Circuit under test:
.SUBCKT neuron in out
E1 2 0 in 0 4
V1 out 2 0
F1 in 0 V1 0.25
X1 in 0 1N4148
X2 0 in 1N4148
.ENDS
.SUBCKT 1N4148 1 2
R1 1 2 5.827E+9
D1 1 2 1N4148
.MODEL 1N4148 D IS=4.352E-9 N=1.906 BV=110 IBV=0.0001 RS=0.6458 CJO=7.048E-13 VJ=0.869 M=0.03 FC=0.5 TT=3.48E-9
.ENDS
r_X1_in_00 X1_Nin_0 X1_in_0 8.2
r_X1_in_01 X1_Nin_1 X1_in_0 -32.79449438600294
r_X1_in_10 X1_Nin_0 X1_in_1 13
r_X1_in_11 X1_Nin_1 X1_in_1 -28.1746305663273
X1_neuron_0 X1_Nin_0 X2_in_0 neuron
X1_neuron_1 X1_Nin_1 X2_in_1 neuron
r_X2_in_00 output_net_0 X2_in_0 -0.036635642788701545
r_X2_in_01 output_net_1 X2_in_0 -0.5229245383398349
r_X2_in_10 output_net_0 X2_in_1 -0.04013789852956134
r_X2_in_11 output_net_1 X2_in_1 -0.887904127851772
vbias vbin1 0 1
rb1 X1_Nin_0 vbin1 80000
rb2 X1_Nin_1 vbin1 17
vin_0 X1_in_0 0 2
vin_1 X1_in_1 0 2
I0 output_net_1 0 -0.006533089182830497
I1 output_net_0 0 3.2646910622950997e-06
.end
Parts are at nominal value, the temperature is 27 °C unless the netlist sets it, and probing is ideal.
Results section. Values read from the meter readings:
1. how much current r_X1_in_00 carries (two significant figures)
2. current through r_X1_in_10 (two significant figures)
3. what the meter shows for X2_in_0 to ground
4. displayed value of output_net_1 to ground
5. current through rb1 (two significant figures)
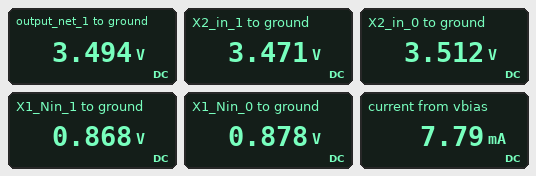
140 mA
86 mA
3.512 V
3.494 V
1.5 µA
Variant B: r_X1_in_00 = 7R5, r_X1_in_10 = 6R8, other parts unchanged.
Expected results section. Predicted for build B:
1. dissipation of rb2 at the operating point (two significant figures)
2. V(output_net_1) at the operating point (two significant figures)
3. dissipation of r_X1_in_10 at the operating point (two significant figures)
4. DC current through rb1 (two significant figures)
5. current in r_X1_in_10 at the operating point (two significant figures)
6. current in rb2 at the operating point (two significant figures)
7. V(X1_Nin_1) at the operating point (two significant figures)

460 µW
3.7 V
170 mW
940 nA
160 mA
5.2 mA
910 mV
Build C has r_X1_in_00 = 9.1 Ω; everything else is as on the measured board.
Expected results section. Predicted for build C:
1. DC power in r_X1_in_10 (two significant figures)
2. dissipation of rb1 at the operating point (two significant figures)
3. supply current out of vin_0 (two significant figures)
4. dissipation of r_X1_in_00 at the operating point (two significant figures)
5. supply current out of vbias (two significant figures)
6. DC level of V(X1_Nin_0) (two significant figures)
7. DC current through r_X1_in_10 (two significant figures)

98 mW
210 nW
89 mA
140 mW
8.2 mA
870 mV
87 mA
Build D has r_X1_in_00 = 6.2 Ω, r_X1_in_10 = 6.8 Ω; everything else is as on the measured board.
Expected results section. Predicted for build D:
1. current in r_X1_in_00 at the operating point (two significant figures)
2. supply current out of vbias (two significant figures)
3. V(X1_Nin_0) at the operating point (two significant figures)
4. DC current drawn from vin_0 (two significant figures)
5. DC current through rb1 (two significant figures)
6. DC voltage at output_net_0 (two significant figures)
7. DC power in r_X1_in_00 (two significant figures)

170 mA
4.4 mA
940 mV
140 mA
760 nA
3.7 V
180 mW
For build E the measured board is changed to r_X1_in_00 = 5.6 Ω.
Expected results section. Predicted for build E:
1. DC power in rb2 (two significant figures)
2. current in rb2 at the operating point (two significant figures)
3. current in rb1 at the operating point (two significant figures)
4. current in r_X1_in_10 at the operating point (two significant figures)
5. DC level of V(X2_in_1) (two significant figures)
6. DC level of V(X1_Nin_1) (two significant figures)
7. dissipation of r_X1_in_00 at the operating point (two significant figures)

590 µW
5.9 mA
1.1 µA
84 mA
3.6 V
900 mV
210 mW
